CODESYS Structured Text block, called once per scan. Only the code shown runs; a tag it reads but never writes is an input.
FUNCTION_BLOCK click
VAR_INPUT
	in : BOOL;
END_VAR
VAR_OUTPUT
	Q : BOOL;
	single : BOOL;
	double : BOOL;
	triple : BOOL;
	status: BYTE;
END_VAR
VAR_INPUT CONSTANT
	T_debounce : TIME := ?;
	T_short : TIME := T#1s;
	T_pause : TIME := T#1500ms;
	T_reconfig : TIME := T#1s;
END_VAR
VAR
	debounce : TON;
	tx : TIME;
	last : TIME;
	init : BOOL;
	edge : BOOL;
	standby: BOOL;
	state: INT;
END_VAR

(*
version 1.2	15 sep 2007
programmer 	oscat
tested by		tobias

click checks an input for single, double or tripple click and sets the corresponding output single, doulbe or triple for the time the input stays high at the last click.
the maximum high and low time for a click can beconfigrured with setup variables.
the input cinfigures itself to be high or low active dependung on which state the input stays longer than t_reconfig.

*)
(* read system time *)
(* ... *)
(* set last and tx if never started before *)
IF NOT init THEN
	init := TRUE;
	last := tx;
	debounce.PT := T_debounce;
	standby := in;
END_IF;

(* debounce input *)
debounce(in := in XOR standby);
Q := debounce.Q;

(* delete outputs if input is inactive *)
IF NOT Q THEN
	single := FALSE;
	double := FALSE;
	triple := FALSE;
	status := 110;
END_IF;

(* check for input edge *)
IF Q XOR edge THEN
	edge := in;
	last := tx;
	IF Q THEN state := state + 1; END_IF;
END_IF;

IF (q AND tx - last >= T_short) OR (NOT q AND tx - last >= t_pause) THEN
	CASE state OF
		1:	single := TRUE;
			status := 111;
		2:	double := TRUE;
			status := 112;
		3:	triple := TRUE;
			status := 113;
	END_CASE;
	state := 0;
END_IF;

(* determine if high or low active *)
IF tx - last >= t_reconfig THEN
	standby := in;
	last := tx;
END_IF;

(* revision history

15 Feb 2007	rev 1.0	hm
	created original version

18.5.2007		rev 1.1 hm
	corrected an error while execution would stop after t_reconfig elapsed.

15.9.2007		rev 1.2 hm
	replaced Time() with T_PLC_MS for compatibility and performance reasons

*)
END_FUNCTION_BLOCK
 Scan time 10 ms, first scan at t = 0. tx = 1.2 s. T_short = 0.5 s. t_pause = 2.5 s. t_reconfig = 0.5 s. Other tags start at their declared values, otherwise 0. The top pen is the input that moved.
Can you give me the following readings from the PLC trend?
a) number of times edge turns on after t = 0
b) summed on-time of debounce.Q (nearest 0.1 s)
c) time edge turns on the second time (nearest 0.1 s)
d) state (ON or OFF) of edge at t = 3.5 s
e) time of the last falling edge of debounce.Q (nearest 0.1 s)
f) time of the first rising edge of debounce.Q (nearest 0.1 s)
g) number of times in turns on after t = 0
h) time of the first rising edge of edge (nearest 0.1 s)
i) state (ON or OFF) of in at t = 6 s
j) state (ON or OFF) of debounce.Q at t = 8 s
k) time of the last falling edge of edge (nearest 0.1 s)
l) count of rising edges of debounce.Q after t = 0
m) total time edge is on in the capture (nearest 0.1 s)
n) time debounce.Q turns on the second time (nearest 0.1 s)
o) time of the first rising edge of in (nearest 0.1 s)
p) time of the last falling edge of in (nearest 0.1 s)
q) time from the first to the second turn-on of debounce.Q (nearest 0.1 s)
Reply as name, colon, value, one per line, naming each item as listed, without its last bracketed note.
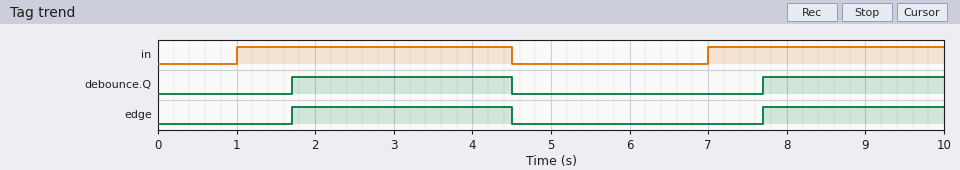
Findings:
number of times edge turns on after t = 0: 2
summed on-time of debounce.Q: 5.1 s
time edge turns on the second time: 7.7 s
state (ON or OFF) of edge at t = 3.5 s: ON
time of the last falling edge of debounce.Q: 4.5 s
time of the first rising edge of debounce.Q: 1.7 s
number of times in turns on after t = 0: 2
time of the first rising edge of edge: 1.7 s
state (ON or OFF) of in at t = 6 s: OFF
state (ON or OFF) of debounce.Q at t = 8 s: ON
time of the last falling edge of edge: 4.5 s
count of rising edges of debounce.Q after t = 0: 2
total time edge is on in the capture: 5.1 s
time debounce.Q turns on the second time: 7.7 s
time of the first rising edge of in: 1.0 s
time of the last falling edge of in: 4.5 s
time from the first to the second turn-on of debounce.Q: 6.0 s
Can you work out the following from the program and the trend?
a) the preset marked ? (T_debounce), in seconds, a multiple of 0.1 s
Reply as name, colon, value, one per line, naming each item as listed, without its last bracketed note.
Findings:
the preset marked ? (T_debounce), in seconds, a multiple of 0.1 s: 0.7 s
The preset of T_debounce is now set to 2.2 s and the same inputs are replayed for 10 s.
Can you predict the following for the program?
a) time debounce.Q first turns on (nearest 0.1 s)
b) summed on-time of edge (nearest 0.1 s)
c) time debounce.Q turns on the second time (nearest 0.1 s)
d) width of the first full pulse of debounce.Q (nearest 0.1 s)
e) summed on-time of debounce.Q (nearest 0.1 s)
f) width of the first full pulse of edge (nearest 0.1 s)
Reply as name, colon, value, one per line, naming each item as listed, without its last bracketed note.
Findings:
time debounce.Q first turns on: 3.2 s
summed on-time of edge: 2.1 s
time debounce.Q turns on the second time: 9.2 s
width of the first full pulse of debounce.Q: 1.3 s
summed on-time of debounce.Q: 2.1 s
width of the first full pulse of edge: 1.3 s
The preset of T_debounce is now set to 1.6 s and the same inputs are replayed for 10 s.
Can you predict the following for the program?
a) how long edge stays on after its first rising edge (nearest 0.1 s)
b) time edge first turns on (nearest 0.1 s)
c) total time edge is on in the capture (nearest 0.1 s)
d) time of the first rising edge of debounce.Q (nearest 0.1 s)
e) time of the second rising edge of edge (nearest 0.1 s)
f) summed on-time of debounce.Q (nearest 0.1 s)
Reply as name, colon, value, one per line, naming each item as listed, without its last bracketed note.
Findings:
how long edge stays on after its first rising edge: 1.9 s
time edge first turns on: 2.6 s
total time edge is on in the capture: 3.3 s
time of the first rising edge of debounce.Q: 2.6 s
time of the second rising edge of edge: 8.6 s
summed on-time of debounce.Q: 3.3 s
